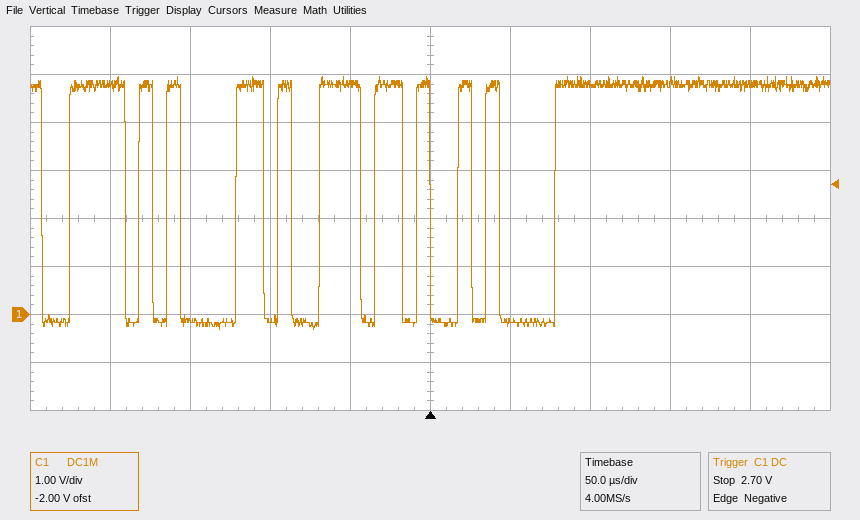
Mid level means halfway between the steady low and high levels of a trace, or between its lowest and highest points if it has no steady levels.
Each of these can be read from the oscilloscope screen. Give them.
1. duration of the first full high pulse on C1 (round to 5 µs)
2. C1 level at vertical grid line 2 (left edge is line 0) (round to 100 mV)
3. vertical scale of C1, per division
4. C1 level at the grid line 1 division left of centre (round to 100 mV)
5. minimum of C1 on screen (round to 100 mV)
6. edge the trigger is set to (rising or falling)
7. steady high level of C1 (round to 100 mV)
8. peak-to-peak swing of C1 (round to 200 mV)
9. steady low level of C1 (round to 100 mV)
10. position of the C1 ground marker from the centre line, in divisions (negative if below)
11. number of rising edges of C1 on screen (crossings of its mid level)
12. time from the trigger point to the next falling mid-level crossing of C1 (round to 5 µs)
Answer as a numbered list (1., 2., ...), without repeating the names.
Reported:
1. 35 µs
2. -100 mV
3. 1 V
4. 4.8 V
5. -300 mV
6. falling
7. 4.8 V
8. 5.2 V
9. -200 mV
10. -2.0 div
11. 11
12. 25 µs
